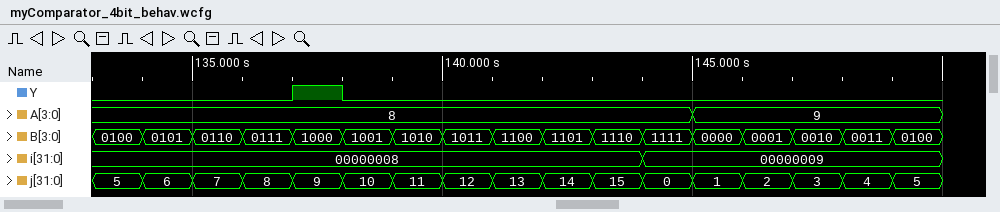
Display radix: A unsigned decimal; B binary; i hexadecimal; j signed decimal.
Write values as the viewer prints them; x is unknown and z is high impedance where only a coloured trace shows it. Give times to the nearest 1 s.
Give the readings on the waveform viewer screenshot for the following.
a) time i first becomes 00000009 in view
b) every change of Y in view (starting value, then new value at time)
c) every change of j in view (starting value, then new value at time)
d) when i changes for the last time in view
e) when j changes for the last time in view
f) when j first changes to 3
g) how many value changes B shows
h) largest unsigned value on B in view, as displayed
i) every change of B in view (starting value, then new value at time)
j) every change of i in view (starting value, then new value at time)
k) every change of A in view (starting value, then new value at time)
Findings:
144 s
0, 1 at 137 s, 0 at 138 s
5, 6 at 134 s, 7 at 135 s, 8 at 136 s, 9 at 137 s, 10 at 138 s, 11 at 139 s, 12 at 140 s, 13 at 141 s, 14 at 142 s, 15 at 143 s, 0 at 144 s, 1 at 145 s, 2 at 146 s, 3 at 147 s, 4 at 148 s, 5 at 149 s
144 s
149 s
147 s
16
1111
0100, 0101 at 134 s, 0110 at 135 s, 0111 at 136 s, 1000 at 137 s, 1001 at 138 s, 1010 at 139 s, 1011 at 140 s, 1100 at 141 s, 1101 at 142 s, 1110 at 143 s, 1111 at 144 s, 0000 at 145 s, 0001 at 146 s, 0010 at 147 s, 0011 at 148 s, 0100 at 149 s
00000008, 00000009 at 144 s
8, 9 at 145 s
